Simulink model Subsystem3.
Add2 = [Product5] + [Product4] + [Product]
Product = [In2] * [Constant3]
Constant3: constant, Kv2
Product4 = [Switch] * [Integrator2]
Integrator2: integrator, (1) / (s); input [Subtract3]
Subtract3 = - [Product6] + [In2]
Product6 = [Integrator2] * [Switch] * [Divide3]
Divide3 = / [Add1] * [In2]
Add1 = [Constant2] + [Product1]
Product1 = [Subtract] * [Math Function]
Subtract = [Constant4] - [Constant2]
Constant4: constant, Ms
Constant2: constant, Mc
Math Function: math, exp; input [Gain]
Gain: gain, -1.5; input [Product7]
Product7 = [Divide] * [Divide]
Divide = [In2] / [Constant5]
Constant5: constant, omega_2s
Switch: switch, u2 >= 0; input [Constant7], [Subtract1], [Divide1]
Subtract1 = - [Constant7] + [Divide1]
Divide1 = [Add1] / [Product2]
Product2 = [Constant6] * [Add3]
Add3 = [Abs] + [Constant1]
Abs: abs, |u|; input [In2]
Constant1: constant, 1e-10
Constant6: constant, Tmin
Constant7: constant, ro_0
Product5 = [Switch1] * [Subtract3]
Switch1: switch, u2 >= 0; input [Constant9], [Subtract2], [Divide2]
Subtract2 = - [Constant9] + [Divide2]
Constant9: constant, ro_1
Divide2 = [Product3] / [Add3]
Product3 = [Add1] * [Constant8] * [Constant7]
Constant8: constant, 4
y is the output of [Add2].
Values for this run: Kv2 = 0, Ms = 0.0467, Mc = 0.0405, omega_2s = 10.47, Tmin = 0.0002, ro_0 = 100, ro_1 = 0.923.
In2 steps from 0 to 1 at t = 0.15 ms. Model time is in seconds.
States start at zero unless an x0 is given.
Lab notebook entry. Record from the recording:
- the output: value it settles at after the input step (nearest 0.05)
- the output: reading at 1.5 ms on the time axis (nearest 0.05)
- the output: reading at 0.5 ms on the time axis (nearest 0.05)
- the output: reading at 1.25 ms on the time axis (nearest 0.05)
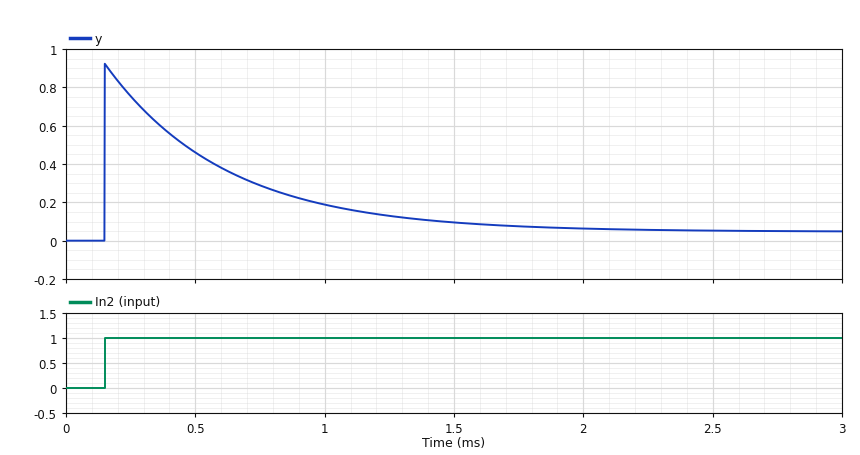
0.05
0.10
0.45
0.15
